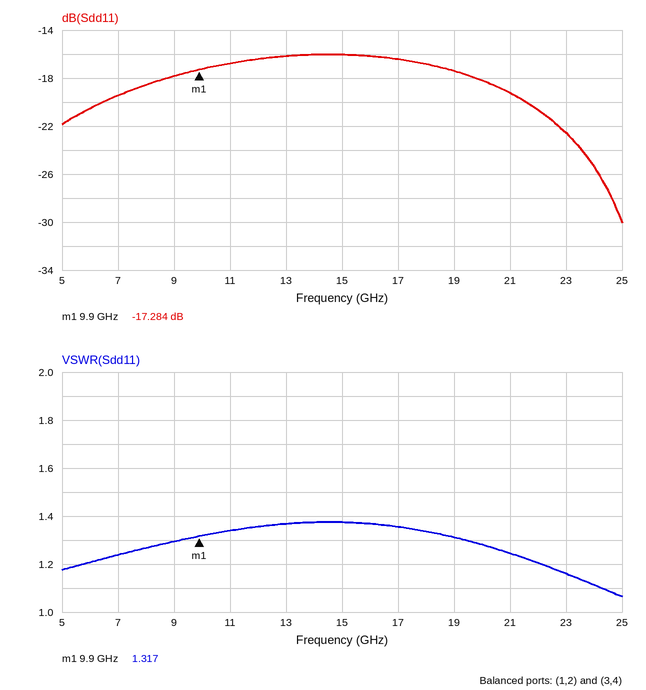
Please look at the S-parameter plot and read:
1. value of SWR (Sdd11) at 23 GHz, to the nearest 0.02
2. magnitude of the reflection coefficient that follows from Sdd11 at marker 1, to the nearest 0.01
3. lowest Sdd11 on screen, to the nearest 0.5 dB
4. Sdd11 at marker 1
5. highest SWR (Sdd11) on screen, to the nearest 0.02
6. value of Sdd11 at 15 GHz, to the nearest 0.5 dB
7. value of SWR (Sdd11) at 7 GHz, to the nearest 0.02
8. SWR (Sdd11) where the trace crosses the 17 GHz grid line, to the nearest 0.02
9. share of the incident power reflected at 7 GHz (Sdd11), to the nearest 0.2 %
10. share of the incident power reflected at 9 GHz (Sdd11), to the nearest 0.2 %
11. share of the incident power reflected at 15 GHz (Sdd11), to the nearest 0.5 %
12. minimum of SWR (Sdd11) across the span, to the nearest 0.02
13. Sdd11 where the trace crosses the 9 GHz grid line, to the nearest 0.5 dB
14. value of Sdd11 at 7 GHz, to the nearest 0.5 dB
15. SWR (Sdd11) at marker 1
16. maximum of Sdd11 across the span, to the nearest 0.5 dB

1.16
0.14
-30.0 dB
-17.284 dB
1.38
-16.0 dB
1.24
1.36
1.2 %
1.6 %
2.5 %
1.06
-18.0 dB
-19.5 dB
1.317
-16.0 dB
